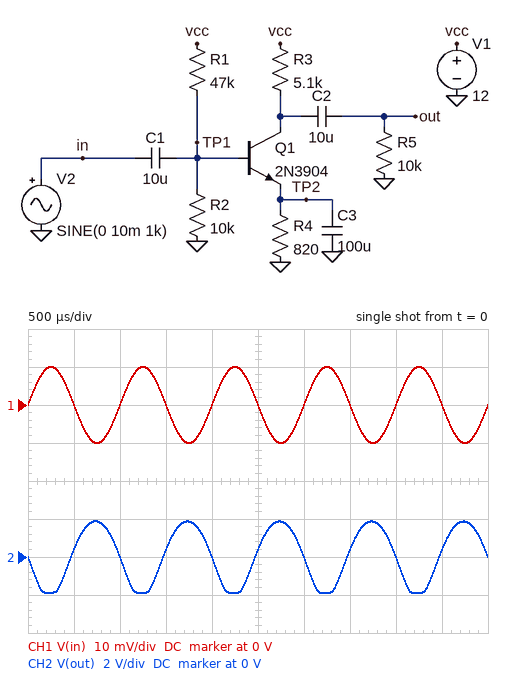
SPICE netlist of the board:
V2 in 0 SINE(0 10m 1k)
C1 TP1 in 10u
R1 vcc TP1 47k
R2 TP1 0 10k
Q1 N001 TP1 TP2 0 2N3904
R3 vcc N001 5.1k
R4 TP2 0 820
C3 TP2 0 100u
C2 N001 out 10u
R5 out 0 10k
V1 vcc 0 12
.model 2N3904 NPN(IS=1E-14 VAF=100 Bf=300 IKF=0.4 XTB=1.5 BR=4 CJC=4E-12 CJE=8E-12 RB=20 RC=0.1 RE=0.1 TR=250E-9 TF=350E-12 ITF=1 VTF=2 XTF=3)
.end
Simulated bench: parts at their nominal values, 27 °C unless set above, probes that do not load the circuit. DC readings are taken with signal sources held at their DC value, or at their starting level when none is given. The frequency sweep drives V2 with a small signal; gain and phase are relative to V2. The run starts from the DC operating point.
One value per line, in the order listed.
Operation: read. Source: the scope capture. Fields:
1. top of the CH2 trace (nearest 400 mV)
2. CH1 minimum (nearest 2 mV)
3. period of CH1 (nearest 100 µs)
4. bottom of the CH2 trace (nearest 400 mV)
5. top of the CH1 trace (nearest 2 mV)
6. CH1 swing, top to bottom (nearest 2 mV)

2.0 V
-10 mV
1.0 ms
-2.0 V
10 mV
20 mV
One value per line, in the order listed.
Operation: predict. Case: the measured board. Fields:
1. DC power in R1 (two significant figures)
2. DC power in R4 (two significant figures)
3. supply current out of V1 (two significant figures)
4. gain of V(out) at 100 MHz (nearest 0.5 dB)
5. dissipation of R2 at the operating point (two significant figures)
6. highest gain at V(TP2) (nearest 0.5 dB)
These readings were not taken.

2.1 mW
2.4 mW
1.9 mA
23.5 dB
420 µW
-0.5 dB
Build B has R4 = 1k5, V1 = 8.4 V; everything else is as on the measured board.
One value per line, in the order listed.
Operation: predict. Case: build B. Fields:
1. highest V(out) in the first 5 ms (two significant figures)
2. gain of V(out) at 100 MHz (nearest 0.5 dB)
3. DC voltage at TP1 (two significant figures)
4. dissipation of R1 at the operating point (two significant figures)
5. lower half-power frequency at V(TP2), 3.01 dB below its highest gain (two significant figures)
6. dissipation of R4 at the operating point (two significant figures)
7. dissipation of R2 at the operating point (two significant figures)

620 mV
20.5 dB
1.5 V
1.0 mW
1.7 Hz
450 µW
210 µW
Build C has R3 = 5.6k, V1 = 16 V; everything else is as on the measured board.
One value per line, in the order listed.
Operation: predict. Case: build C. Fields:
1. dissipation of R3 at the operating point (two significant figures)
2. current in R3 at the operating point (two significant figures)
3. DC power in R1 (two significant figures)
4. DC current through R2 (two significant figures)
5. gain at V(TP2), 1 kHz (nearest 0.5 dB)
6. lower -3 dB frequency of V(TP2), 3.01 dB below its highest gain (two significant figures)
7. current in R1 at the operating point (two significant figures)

34 mW
2.5 mA
3.8 mW
270 µA
-25.5 dB
2.5 Hz
280 µA
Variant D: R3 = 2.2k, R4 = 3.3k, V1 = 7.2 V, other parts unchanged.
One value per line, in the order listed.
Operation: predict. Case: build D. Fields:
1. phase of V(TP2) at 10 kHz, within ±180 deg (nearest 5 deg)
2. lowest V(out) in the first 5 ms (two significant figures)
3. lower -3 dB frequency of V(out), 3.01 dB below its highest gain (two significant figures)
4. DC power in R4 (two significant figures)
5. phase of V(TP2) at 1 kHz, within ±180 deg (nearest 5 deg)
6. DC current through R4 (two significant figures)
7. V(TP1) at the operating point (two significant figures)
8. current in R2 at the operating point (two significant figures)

-90 deg
-160 mV
13 Hz
130 µW
-90 deg
200 µA
1.3 V
130 µA
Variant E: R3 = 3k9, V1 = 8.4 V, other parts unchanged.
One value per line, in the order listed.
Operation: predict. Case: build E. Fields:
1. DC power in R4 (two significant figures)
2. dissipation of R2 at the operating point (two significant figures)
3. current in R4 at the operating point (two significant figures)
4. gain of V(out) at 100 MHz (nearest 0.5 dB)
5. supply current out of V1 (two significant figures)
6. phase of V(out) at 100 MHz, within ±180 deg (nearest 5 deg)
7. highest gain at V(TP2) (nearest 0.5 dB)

770 µW
210 µW
970 µA
23.0 dB
1.1 mA
85 deg
-1.0 dB
